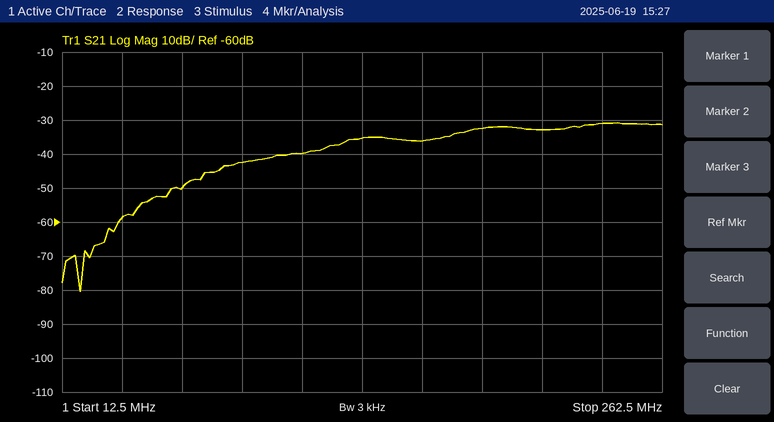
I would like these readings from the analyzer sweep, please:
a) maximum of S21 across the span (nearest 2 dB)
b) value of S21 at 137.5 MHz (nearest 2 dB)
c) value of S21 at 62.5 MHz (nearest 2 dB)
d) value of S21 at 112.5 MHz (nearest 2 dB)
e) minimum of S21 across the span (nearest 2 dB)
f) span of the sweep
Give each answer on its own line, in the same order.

-30 dB
-36 dB
-50 dB
-40 dB
-80 dB
250 MHz
